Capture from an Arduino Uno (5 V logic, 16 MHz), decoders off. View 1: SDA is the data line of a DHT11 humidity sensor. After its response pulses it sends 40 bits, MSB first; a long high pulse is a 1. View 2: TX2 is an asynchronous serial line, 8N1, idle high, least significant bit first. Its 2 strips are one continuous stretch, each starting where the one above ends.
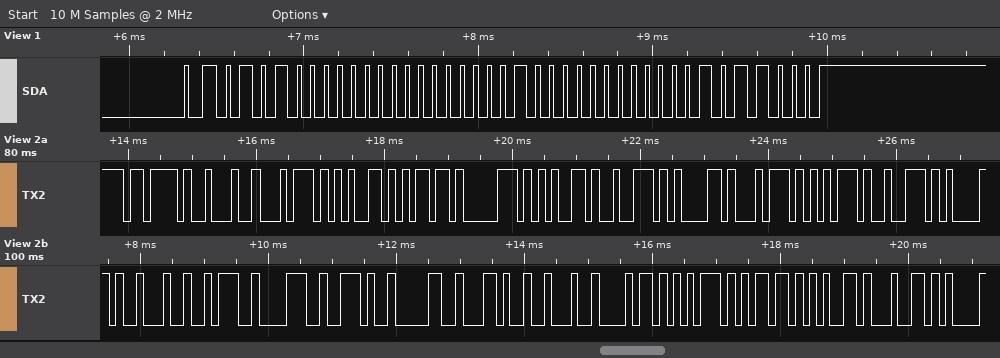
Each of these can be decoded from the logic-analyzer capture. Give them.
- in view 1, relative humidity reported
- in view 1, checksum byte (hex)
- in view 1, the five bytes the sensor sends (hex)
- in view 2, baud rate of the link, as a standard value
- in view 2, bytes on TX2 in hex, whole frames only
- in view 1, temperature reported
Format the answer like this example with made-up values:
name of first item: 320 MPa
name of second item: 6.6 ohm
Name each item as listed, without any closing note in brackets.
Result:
in view 1, relative humidity reported: 80 %
in view 1, checksum byte: 0x58
in view 1, the five bytes the sensor sends: 50 00 08 00 58
in view 2, baud rate of the link, as a standard value: 9600 baud
in view 2, bytes on TX2 in hex, whole frames only: 0x7B 0x22 0x74 0x65 0x6D 0x70 0x65 0x72 0x61 0x74 0x75 0x72 0x61 0x22 0x3A 0x38 0x2E 0x30 0x2C 0x22 0x68 0x75 0x6D 0x65 0x64
in view 1, temperature reported: 8.0 °C
